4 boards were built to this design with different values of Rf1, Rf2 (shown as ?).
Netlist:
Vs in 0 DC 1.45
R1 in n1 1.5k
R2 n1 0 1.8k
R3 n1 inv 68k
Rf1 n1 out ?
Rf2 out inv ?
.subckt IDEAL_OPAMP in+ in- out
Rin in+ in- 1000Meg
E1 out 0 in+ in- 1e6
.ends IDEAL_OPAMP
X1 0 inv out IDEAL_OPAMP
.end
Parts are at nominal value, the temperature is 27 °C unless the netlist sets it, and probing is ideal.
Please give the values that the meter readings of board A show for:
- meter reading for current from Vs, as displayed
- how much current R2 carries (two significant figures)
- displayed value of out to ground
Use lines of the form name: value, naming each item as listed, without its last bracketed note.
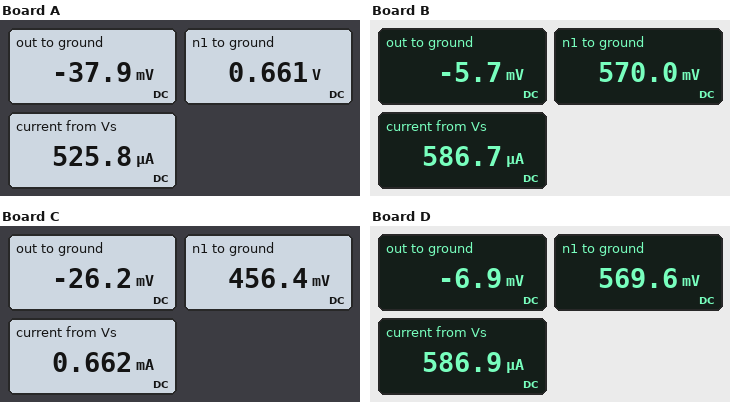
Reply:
meter reading for current from Vs, as displayed: 525.8 µA
how much current R2 carries: 370 µA
displayed value of out to ground: -37.9 mV
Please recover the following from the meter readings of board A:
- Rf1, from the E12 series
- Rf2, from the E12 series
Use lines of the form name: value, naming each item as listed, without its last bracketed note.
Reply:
Rf1, from the E12 series: 4.7 kΩ
Rf2, from the E12 series: 3.9 kΩ
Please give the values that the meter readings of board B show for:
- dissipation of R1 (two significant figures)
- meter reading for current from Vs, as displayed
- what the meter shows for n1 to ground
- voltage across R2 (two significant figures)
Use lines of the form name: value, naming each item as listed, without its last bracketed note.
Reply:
dissipation of R1: 520 µW
meter reading for current from Vs, as displayed: 586.7 µA
what the meter shows for n1 to ground: 570.0 mV
voltage across R2: 570 mV
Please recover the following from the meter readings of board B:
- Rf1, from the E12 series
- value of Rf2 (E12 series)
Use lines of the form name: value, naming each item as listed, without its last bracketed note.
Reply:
Rf1, from the E12 series: 2.2 kΩ
value of Rf2: 680 Ω
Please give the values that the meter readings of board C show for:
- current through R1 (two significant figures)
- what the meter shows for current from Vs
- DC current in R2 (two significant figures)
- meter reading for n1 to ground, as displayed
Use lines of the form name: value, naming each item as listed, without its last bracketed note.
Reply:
current through R1: 660 µA
what the meter shows for current from Vs: 0.662 mA
DC current in R2: 250 µA
meter reading for n1 to ground, as displayed: 456.4 mV
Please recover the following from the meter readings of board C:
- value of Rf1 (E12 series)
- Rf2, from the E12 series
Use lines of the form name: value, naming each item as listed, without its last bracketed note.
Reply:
value of Rf1: 1.2 kΩ
Rf2, from the E12 series: 3.9 kΩ
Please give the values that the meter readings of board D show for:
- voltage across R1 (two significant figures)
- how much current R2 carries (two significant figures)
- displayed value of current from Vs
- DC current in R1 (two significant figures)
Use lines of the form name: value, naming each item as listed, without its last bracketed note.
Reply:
voltage across R1: 880 mV
how much current R2 carries: 320 µA
displayed value of current from Vs: 586.9 µA
DC current in R1: 590 µA
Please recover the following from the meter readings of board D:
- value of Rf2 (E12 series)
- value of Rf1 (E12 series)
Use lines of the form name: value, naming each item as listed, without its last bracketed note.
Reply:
value of Rf2: 820 Ω
value of Rf1: 2.2 kΩ
